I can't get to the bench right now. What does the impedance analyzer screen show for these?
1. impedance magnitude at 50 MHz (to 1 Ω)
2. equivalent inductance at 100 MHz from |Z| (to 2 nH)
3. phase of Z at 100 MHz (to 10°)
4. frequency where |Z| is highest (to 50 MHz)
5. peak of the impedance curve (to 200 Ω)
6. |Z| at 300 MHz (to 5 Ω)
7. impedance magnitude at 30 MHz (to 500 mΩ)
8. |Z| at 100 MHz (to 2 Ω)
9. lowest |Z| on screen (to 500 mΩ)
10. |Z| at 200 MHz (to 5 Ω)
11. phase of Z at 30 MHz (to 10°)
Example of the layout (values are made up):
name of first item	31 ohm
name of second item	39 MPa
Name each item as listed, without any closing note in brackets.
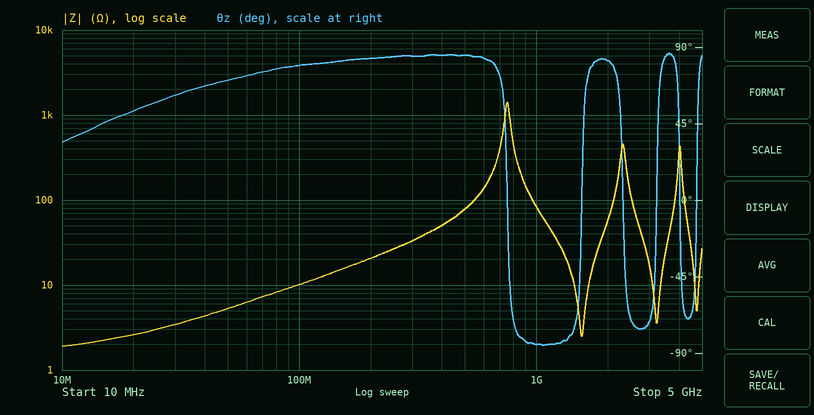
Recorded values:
impedance magnitude at 50 MHz	5 Ω
equivalent inductance at 100 MHz from |Z|	16 nH
phase of Z at 100 MHz	80°
frequency where |Z| is highest	750 MHz
peak of the impedance curve	1.4 kΩ
|Z| at 300 MHz	35 Ω
impedance magnitude at 30 MHz	3.5 Ω
|Z| at 100 MHz	10 Ω
lowest |Z| on screen	2.0 Ω
|Z| at 200 MHz	20 Ω
phase of Z at 30 MHz	60°
